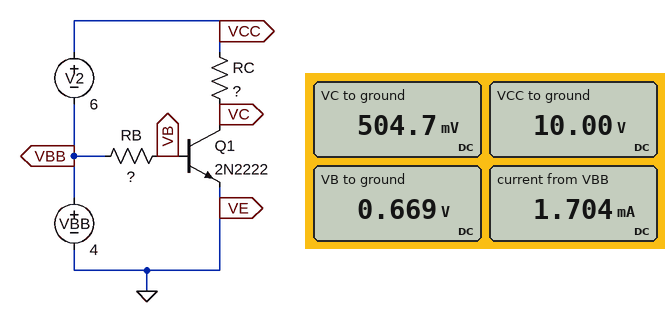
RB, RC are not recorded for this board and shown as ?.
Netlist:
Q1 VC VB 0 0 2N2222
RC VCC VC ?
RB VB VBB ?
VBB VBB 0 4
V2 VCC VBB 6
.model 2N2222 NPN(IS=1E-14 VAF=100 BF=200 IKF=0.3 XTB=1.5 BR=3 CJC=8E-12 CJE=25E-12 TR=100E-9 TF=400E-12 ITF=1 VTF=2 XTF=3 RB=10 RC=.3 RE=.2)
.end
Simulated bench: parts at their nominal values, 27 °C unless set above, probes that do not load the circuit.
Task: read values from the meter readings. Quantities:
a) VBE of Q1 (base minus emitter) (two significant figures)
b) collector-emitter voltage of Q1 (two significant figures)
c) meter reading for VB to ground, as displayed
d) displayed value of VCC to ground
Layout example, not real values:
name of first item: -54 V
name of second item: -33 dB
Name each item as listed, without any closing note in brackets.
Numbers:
VBE of Q1 (base minus emitter): 670 mV
collector-emitter voltage of Q1: 500 mV
meter reading for VB to ground, as displayed: 0.669 V
displayed value of VCC to ground: 10.00 V
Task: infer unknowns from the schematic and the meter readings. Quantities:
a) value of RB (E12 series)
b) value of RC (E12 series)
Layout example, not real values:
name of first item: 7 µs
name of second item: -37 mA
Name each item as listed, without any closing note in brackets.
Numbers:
value of RB: 390 kΩ
value of RC: 5.6 kΩ
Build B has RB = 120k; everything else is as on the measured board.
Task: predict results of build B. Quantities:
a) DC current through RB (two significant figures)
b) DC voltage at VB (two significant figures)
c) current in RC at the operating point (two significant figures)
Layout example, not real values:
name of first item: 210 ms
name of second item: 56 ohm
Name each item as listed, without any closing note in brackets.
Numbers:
DC current through RB: 28 µA
DC voltage at VB: 670 mV
current in RC at the operating point: 1.8 mA
